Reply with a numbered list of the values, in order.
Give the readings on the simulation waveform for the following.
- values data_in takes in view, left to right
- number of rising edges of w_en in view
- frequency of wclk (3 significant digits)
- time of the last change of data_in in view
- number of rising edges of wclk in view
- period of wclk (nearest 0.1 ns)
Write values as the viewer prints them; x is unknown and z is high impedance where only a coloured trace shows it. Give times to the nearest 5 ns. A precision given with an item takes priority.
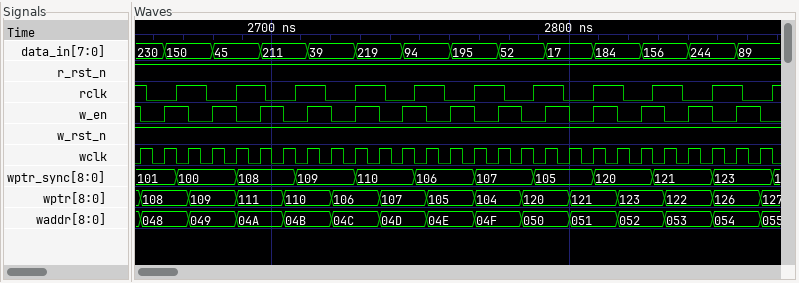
1. 230, 150, 45, 211, 39, 219, 94, 195, 52, 17, 184, 156, 244, 89
2. 13
3. 125 MHz
4. 2855 ns
5. 27
6. 8 ns
